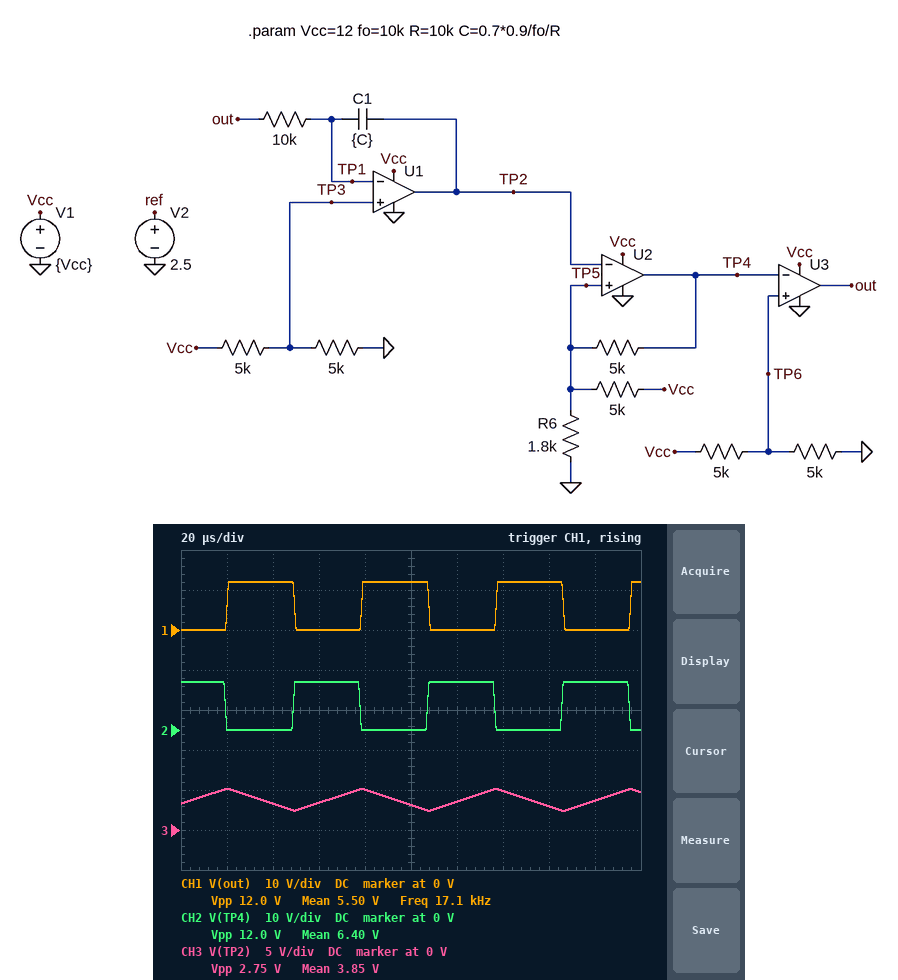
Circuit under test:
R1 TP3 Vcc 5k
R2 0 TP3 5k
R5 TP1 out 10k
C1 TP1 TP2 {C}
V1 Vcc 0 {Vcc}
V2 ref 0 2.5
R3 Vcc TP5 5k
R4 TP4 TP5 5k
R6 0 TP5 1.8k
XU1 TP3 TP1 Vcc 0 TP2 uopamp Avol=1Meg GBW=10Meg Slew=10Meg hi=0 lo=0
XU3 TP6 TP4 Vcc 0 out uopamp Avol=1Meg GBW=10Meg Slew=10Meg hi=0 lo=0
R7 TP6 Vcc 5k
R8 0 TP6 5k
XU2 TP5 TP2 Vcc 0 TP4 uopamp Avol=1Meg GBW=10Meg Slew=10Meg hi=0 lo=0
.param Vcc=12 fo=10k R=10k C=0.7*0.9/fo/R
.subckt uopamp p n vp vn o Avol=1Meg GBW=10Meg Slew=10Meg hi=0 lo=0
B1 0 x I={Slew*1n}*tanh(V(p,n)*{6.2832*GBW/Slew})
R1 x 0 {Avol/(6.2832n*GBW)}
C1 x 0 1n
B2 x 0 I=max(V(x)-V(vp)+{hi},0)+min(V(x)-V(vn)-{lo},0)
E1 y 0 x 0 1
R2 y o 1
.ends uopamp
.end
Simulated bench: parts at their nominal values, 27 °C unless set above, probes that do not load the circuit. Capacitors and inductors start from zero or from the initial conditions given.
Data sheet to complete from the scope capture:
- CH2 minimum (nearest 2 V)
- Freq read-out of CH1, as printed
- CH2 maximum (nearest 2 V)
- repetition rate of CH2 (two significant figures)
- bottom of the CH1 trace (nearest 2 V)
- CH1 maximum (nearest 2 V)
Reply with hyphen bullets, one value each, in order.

- 0 V
- 17.1 kHz
- 12 V
- 17 kHz
- 0 V
- 12 V
